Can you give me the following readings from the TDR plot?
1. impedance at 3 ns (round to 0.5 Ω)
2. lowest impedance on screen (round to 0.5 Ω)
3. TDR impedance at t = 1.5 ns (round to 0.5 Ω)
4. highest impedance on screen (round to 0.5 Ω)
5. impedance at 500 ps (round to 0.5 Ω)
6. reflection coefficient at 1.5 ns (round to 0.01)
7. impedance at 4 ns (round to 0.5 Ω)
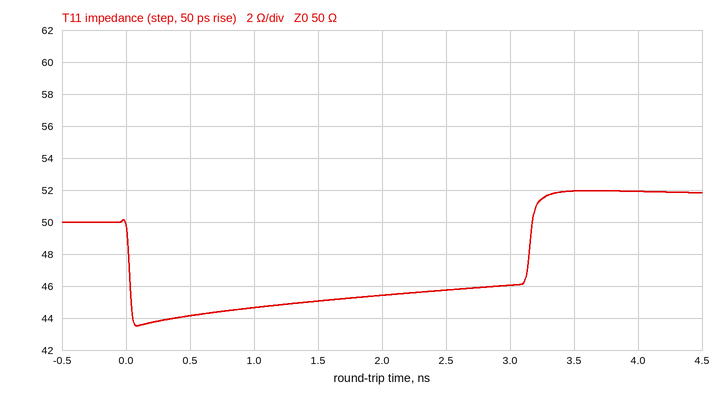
46.0 Ω
43.5 Ω
45.0 Ω
52.0 Ω
44.0 Ω
-0.05
52.0 Ω
